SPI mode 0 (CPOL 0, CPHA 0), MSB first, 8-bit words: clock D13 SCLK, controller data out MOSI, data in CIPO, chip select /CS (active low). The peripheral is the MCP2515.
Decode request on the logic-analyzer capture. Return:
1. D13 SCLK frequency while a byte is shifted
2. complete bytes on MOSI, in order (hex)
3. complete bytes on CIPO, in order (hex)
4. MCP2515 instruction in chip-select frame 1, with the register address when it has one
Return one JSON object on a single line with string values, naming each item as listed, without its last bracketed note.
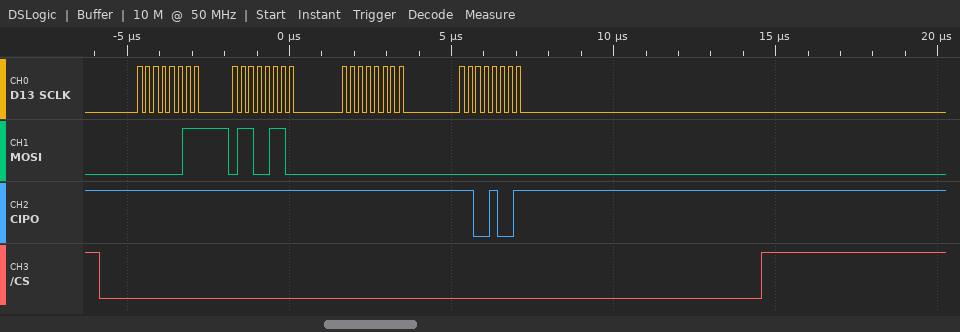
{"D13 SCLK frequency while a byte is shifted": "4 MHz", "complete bytes on MOSI, in order": "03 66 00 00", "complete bytes on CIPO, in order": "FF FF FF C9", "MCP2515 instruction in chip-select frame 1, with the register address when it has one": "READ 0x66"}
